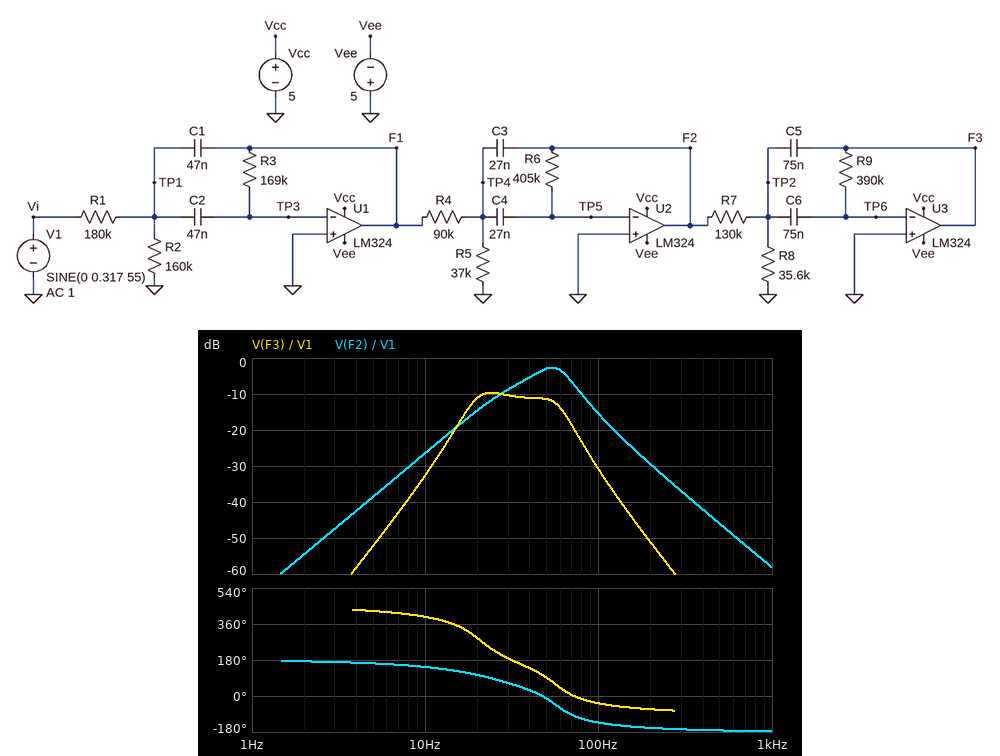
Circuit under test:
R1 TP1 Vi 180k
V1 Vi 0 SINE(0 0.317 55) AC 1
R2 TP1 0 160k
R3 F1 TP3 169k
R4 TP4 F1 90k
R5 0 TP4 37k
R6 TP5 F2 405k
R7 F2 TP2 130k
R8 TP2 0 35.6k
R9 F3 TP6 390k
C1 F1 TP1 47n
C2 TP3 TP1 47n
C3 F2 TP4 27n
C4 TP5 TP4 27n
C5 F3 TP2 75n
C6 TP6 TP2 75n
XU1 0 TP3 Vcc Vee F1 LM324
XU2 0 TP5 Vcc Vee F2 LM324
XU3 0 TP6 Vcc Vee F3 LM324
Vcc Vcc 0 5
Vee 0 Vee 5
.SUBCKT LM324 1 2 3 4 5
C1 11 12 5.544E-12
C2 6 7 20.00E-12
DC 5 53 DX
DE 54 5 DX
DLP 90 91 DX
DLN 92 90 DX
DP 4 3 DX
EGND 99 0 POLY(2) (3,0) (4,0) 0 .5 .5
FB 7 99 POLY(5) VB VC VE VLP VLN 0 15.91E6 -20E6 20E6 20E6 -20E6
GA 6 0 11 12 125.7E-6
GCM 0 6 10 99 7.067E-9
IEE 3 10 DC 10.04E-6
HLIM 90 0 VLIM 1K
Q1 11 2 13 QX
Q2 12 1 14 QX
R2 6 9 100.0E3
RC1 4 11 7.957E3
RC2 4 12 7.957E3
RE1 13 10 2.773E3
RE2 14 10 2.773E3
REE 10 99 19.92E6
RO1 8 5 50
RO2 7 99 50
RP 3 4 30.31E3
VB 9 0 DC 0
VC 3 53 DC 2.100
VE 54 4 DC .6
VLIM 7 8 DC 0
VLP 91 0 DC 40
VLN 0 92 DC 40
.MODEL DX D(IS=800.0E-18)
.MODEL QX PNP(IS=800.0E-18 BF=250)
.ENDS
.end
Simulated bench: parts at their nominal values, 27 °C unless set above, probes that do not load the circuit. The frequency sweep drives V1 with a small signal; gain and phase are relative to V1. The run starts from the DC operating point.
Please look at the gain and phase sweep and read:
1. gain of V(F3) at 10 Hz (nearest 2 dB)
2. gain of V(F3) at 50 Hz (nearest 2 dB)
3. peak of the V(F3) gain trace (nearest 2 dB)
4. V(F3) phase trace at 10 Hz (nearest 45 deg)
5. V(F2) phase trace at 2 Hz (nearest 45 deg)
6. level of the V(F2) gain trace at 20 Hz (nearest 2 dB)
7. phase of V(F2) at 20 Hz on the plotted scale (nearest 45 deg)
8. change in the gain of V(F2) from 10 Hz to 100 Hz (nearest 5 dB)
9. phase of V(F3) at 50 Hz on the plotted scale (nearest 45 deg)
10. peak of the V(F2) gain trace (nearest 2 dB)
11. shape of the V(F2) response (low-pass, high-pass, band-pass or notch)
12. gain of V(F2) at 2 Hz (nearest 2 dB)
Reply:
-32 dB
-12 dB
-10 dB
405 deg
180 deg
-14 dB
90 deg
10 dB
90 deg
-2 dB
band-pass
-54 dB
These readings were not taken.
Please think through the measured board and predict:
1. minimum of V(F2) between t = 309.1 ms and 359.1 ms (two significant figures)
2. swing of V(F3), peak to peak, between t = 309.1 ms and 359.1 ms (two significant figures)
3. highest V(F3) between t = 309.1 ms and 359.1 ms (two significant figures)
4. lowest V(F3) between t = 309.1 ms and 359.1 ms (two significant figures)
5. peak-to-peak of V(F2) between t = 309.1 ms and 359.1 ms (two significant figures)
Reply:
-240 mV
160 mV
70 mV
-86 mV
470 mV
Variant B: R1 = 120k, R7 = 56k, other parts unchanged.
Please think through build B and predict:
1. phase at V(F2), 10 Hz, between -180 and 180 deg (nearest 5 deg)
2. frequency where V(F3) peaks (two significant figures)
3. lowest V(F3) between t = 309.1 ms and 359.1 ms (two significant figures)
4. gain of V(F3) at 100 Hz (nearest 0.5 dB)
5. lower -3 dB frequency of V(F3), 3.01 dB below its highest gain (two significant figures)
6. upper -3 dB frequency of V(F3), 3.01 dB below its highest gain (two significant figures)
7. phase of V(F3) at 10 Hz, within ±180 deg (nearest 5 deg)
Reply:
150 deg
26 Hz
-300 mV
-20.0 dB
21 Hz
55 Hz
45 deg
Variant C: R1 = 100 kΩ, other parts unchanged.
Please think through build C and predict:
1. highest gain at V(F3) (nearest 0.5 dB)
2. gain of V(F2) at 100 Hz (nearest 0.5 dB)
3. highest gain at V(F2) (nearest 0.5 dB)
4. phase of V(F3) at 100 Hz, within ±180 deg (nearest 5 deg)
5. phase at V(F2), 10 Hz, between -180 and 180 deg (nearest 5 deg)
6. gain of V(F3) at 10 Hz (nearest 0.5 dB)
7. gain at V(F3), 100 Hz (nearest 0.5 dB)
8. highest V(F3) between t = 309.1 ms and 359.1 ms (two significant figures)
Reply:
-5.5 dB
-10.0 dB
3.0 dB
-35 deg
155 deg
-30.0 dB
-25.5 dB
140 mV
